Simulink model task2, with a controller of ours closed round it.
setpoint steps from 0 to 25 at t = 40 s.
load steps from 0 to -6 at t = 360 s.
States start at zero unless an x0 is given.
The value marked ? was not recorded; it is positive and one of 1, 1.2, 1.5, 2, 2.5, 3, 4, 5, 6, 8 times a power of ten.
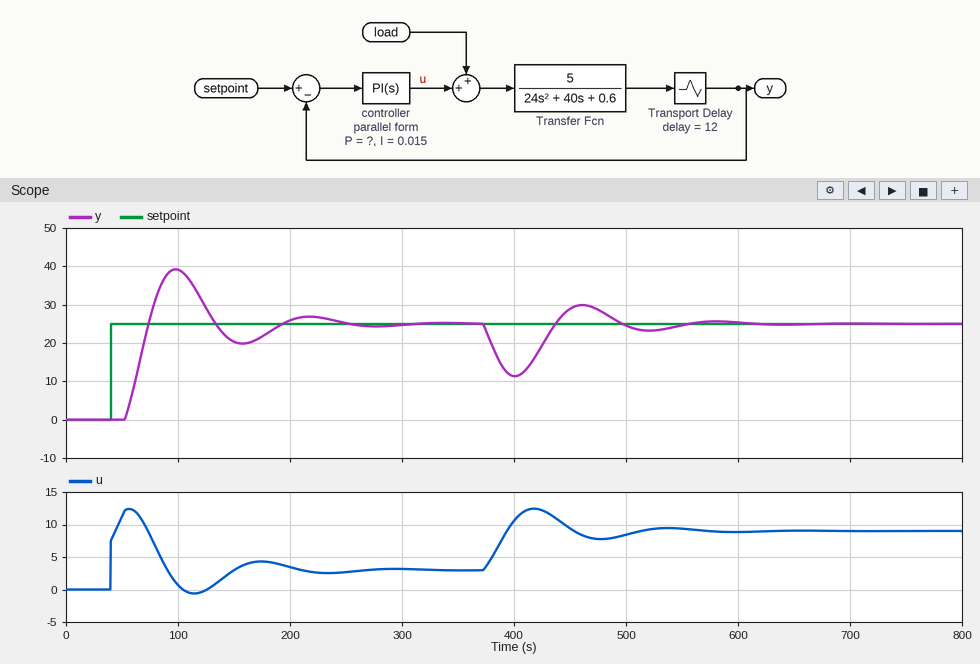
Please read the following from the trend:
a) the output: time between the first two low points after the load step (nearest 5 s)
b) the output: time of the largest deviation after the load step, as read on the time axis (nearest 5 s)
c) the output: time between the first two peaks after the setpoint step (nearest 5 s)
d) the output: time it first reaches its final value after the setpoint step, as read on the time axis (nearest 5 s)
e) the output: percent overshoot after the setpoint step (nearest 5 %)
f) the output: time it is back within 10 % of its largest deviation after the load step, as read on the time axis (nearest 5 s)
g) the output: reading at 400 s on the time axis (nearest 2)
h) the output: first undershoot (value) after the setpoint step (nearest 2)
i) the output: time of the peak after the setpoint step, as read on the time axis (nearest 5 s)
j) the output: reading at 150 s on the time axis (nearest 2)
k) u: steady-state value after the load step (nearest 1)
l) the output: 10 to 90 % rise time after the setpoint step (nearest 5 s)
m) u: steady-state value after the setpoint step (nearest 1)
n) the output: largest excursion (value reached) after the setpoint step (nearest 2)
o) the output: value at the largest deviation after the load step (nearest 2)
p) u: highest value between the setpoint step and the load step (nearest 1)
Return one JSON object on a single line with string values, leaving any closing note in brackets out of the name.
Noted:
{"the output: time between the first two low points after the load step": "120 s", "the output: time of the largest deviation after the load step, as read on the time axis": "400 s", "the output: time between the first two peaks after the setpoint step": "120 s", "the output: time it first reaches its final value after the setpoint step, as read on the time axis": "75 s", "the output: percent overshoot after the setpoint step": "55 %", "the output: time it is back within 10 % of its largest deviation after the load step, as read on the time axis": "535 s", "the output: reading at 400 s on the time axis": "12", "the output: first undershoot (value) after the setpoint step": "20", "the output: time of the peak after the setpoint step, as read on the time axis": "100 s", "the output: reading at 150 s on the time axis": "20", "u: steady-state value after the load step": "9", "the output: 10 to 90 % rise time after the setpoint step": "15 s", "u: steady-state value after the setpoint step": "3", "the output: largest excursion (value reached) after the setpoint step": "40", "the output: value at the largest deviation after the load step": "12", "u: highest value between the setpoint step and the load step": "12"}
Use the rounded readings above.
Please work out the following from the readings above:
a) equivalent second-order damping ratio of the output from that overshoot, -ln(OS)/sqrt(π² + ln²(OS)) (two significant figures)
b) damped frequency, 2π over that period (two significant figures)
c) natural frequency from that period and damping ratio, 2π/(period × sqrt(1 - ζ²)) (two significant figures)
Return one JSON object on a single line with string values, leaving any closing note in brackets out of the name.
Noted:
{"equivalent second-order damping ratio of the output from that overshoot, -ln(OS)/sqrt(π² + ln²(OS))": "0.19", "damped frequency, 2π over that period": "0.052 rad/s", "natural frequency from that period and damping ratio, 2π/(period × sqrt(1 - ζ²))": "0.053 rad/s"}
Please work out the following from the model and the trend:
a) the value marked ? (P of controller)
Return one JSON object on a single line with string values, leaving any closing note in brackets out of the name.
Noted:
{"the value marked ?": "0.3"}
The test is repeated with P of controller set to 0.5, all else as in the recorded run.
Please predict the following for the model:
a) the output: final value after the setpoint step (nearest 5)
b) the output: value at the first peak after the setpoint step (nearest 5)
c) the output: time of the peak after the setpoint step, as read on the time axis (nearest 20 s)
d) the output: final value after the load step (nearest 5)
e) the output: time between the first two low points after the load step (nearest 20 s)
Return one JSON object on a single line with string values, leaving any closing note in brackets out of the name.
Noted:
{"the output: final value after the setpoint step": "25", "the output: value at the first peak after the setpoint step": "40", "the output: time of the peak after the setpoint step, as read on the time axis": "80 s", "the output: final value after the load step": "25", "the output: time between the first two low points after the load step": "80 s"}
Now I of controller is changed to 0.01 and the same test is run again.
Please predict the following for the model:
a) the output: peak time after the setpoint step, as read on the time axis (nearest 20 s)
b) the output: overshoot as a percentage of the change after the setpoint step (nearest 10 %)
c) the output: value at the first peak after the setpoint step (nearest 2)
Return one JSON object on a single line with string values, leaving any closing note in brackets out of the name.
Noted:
{"the output: peak time after the setpoint step, as read on the time axis": "100 s", "the output: overshoot as a percentage of the change after the setpoint step": "30 %", "the output: value at the first peak after the setpoint step": "34"}
